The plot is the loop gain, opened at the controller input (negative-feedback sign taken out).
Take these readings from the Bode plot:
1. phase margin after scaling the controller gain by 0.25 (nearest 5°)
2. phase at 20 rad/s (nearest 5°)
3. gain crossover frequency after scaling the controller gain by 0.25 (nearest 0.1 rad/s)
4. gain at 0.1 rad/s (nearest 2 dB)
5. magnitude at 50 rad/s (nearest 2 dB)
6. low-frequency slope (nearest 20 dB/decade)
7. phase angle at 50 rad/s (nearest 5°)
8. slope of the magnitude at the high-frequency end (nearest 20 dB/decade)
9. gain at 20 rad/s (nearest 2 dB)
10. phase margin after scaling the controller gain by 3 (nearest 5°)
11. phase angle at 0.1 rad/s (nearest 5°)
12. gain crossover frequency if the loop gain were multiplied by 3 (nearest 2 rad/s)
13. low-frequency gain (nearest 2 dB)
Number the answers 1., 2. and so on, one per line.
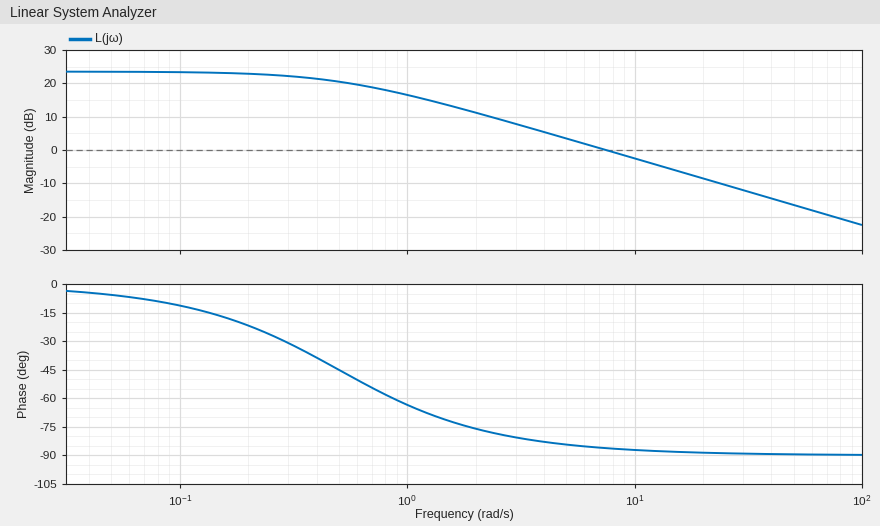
1. 105°
2. -90°
3. 1.8 rad/s
4. 24 dB
5. -16 dB
6. 0 dB/decade
7. -90°
8. -20 dB/decade
9. -8 dB
10. 90°
11. -10°
12. 22 rad/s
13. 24 dB
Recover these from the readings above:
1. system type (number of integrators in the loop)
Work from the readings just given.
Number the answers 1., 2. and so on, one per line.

1. 0
